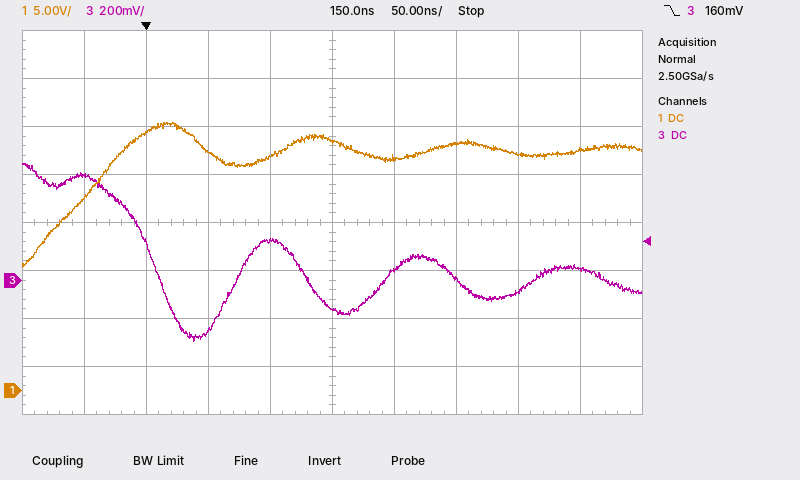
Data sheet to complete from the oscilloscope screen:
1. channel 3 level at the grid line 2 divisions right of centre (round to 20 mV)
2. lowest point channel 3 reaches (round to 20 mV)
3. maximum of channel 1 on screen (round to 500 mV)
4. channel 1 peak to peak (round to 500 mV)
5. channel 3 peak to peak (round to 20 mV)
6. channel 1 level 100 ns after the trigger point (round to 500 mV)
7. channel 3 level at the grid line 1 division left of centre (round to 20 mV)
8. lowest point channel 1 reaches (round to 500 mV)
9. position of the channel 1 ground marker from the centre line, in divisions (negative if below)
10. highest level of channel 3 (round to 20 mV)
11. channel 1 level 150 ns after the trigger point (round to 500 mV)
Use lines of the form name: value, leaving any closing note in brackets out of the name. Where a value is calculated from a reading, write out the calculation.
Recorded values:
channel 3 level at the grid line 2 divisions right of centre: 0 mV
lowest point channel 3 reaches: -260 mV
maximum of channel 1 on screen: 28.0 V
channel 1 peak to peak: 28.0 V − (13.0 V) = 15.0 V
channel 3 peak to peak: 480 mV − (-260 mV) = 740 mV
channel 1 level 100 ns after the trigger point: 24.5 V
channel 3 level at the grid line 1 division left of centre: 160 mV
lowest point channel 1 reaches: 13.0 V
position of the channel 1 ground marker from the centre line, in divisions: -3.5 div
highest level of channel 3: 480 mV
channel 1 level 150 ns after the trigger point: 26.0 V
